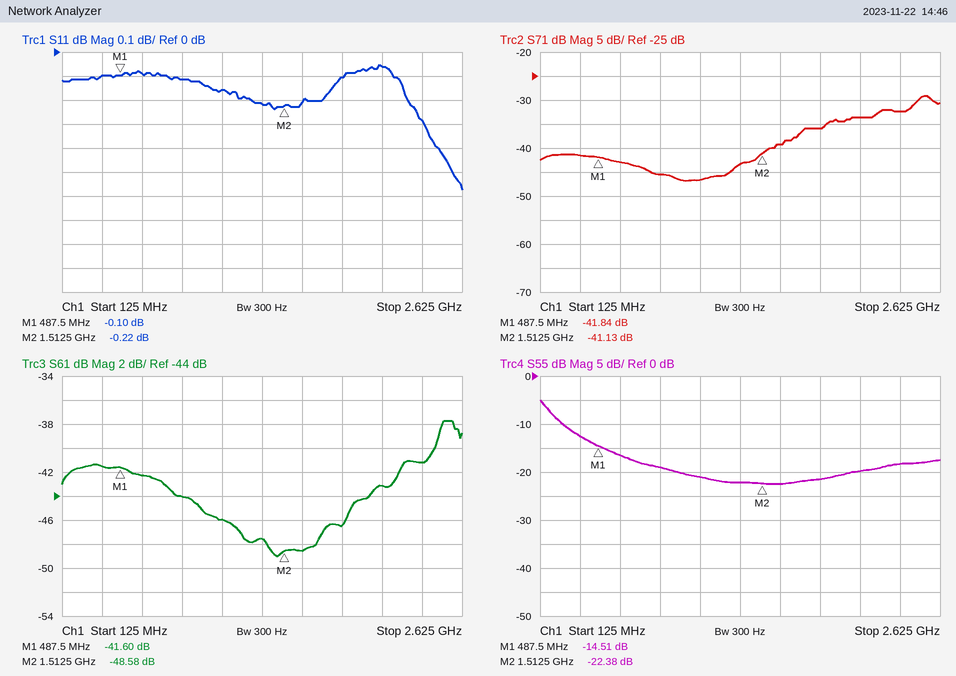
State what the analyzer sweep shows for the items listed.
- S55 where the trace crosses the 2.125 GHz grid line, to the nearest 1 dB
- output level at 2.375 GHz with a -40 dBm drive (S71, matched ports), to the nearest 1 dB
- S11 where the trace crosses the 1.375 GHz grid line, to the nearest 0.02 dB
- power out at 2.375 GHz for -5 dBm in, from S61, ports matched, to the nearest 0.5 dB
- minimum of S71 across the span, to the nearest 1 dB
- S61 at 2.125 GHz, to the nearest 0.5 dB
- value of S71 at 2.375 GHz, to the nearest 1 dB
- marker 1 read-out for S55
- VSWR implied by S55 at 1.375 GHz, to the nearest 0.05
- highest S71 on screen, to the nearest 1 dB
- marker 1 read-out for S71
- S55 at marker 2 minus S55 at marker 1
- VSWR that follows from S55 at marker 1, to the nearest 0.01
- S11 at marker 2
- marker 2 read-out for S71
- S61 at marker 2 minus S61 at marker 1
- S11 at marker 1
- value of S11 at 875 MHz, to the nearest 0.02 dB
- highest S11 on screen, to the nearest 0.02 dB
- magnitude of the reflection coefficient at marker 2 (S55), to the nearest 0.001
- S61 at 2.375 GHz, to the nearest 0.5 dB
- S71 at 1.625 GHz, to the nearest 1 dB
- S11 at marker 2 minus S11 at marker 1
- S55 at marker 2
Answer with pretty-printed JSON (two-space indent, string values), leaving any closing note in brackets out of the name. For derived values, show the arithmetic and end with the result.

{
  "S55 where the trace crosses the 2.125 GHz grid line, to the nearest 1 dB": "-20 dB",
  "output level at 2.375 GHz with a -40 dBm drive (S71, matched ports), to the nearest 1 dB": "-40 dBm + (-32 dB) = -72 dBm",
  "S11 where the trace crosses the 1.375 GHz grid line, to the nearest 0.02 dB": "-0.22 dB",
  "power out at 2.375 GHz for -5 dBm in, from S61, ports matched, to the nearest 0.5 dB": "-5 dBm + (-41.0 dB) = -46.0 dBm",
  "minimum of S71 across the span, to the nearest 1 dB": "-47 dB",
  "S61 at 2.125 GHz, to the nearest 0.5 dB": "-43.0 dB",
  "value of S71 at 2.375 GHz, to the nearest 1 dB": "-32 dB",
  "marker 1 read-out for S55": "-14.51 dB",
  "VSWR implied by S55 at 1.375 GHz, to the nearest 0.05": "|Γ| = 10^(-22/20) = 0.0794; VSWR = (1 + 0.0794)/(1 − 0.0794) ≈ 1.17, so 1.15 to the nearest 0.05",
  "highest S71 on screen, to the nearest 1 dB": "-29 dB",
  "marker 1 read-out for S71": "-41.84 dB",
  "S55 at marker 2 minus S55 at marker 1": "-22.38 − (-14.51) = -7.87 dB",
  "VSWR that follows from S55 at marker 1, to the nearest 0.01": "(1 + 0.1881)/(1 − 0.1881) ≈ 1.46",
  "S11 at marker 2": "-0.22 dB",
  "marker 2 read-out for S71": "-41.13 dB",
  "S61 at marker 2 minus S61 at marker 1": "-48.58 − (-41.6) = -6.98 dB",
  "S11 at marker 1": "-0.10 dB",
  "value of S11 at 875 MHz, to the nearest 0.02 dB": "-0.12 dB",
  "highest S11 on screen, to the nearest 0.02 dB": "-0.06 dB",
  "magnitude of the reflection coefficient at marker 2 (S55), to the nearest 0.001": "10^(-22.38/20) ≈ 0.076",
  "S61 at 2.375 GHz, to the nearest 0.5 dB": "-41.0 dB",
  "S71 at 1.625 GHz, to the nearest 1 dB": "-39 dB",
  "S11 at marker 2 minus S11 at marker 1": "-0.22 − (-0.1) = -0.12 dB",
  "S55 at marker 2": "-22.38 dB"
}
